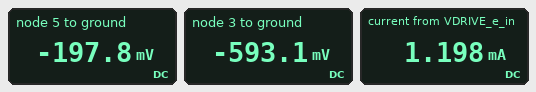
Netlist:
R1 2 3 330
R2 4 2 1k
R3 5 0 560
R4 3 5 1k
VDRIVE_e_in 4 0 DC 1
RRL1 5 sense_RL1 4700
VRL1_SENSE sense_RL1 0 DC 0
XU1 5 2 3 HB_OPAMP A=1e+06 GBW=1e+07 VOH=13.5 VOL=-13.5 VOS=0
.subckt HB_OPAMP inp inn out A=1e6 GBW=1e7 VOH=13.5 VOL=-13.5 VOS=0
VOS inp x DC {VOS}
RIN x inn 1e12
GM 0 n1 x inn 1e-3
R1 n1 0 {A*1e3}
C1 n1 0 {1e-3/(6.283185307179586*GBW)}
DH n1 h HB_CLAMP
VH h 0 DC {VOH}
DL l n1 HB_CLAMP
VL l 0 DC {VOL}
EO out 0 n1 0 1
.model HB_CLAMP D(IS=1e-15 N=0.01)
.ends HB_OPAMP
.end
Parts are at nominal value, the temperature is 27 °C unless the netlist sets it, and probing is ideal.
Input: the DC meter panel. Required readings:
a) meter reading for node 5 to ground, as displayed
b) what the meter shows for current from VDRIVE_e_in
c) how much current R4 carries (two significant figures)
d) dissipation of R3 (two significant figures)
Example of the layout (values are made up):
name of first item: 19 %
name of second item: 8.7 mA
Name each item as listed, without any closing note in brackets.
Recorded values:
meter reading for node 5 to ground, as displayed: -197.8 mV
what the meter shows for current from VDRIVE_e_in: 1.198 mA
how much current R4 carries: 400 µA
dissipation of R3: 70 µW
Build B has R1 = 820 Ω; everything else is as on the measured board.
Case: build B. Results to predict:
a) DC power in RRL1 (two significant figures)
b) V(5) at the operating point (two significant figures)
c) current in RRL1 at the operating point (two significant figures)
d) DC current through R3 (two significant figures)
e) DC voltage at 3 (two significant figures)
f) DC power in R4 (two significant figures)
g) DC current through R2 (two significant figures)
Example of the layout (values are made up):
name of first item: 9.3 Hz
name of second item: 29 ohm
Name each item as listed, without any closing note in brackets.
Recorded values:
DC power in RRL1: 100 µW
V(5) at the operating point: -700 mV
current in RRL1 at the operating point: 150 µA
DC current through R3: 1.2 mA
DC voltage at 3: -2.1 V
DC power in R4: 1.9 mW
DC current through R2: 1.7 mA
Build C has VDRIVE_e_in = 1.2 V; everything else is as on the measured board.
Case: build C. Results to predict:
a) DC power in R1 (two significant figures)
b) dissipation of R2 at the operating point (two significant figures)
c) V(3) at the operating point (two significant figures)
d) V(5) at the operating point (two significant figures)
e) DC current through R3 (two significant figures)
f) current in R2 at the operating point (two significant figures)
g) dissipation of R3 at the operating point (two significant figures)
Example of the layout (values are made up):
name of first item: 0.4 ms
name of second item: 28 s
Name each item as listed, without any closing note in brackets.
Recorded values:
DC power in R1: 680 µW
dissipation of R2 at the operating point: 2.1 mW
V(3) at the operating point: -710 mV
V(5) at the operating point: -240 mV
DC current through R3: 420 µA
current in R2 at the operating point: 1.4 mA
dissipation of R3 at the operating point: 100 µW
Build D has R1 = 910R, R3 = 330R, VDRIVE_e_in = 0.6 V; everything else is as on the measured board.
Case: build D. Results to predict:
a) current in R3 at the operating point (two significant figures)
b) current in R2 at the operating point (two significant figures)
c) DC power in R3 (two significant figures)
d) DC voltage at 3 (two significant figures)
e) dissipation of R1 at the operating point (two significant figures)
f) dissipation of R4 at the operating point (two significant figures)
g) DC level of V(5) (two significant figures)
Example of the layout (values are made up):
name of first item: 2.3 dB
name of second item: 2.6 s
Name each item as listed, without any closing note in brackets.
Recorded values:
current in R3 at the operating point: 710 µA
current in R2 at the operating point: 830 µA
DC power in R3: 170 µW
DC voltage at 3: -990 mV
dissipation of R1 at the operating point: 630 µW
dissipation of R4 at the operating point: 580 µW
DC level of V(5): -230 mV
